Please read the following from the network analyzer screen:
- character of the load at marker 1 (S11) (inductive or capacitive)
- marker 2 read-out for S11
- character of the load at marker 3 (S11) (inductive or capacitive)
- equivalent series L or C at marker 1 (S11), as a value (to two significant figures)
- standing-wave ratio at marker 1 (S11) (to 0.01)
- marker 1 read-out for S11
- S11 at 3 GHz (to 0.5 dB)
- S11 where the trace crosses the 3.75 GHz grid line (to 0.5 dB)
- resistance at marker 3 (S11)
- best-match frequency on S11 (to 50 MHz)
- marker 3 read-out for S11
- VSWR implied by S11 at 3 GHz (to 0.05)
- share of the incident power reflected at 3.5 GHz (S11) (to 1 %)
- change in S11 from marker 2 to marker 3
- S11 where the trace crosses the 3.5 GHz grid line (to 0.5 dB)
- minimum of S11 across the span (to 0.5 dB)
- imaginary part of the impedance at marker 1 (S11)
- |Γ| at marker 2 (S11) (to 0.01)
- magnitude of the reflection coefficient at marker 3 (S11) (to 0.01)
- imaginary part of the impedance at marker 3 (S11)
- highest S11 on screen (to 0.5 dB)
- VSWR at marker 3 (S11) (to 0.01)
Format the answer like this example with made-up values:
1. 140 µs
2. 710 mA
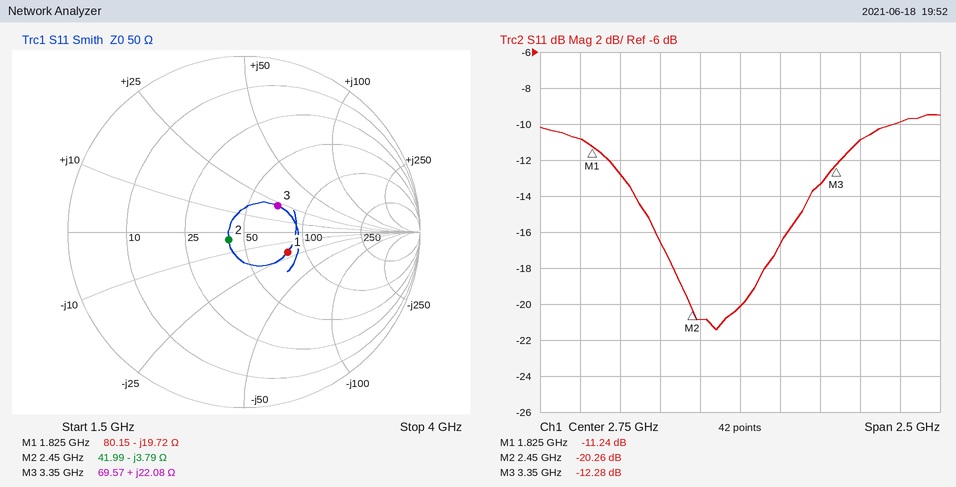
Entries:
1. capacitive
2. -20.26 dB
3. inductive
4. 4.4 pF
5. 1.75
6. -11.24 dB
7. -16.5 dB
8. -10.0 dB
9. 69.57 Ω
10. 2.60 GHz
11. -12.28 dB
12. 1.35
13. 8 %
14. 7.98 dB
15. -11.0 dB
16. -21.5 dB
17. -19.72 Ω
18. 0.10
19. 0.24
20. +22.08 Ω
21. -9.5 dB
22. 1.64
